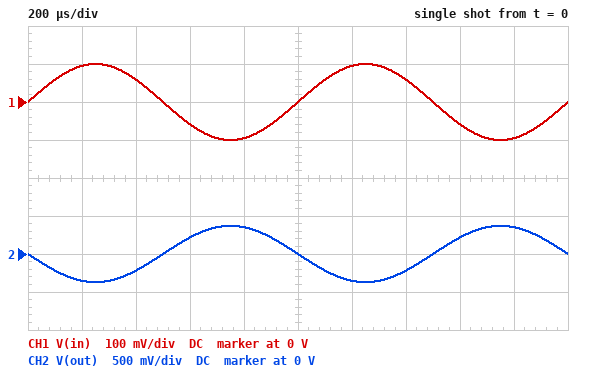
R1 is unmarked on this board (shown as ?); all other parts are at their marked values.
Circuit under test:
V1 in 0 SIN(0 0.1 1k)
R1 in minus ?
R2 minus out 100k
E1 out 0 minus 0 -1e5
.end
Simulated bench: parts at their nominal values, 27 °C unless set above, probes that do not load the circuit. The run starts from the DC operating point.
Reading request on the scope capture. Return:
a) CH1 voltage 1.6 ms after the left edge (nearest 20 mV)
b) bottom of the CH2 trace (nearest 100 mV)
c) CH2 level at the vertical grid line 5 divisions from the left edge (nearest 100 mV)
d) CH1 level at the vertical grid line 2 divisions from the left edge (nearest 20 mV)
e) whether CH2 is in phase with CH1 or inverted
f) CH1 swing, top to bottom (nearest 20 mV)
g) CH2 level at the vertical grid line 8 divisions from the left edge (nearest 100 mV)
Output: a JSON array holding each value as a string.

["-60 mV", "-400 mV", "0 V", "60 mV", "inverted", "200 mV", "200 mV"]
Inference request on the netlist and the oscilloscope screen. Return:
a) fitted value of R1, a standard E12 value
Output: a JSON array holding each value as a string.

["27 kΩ"]
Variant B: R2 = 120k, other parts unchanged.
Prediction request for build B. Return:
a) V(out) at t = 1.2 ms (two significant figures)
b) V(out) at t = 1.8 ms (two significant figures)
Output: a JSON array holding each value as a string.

["-420 mV", "420 mV"]
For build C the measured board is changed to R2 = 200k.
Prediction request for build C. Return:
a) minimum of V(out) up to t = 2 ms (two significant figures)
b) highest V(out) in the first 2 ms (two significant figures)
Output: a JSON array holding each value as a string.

["-740 mV", "740 mV"]
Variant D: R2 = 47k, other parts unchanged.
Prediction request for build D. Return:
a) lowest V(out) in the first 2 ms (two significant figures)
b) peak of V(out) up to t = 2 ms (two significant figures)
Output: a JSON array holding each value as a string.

["-170 mV", "170 mV"]
